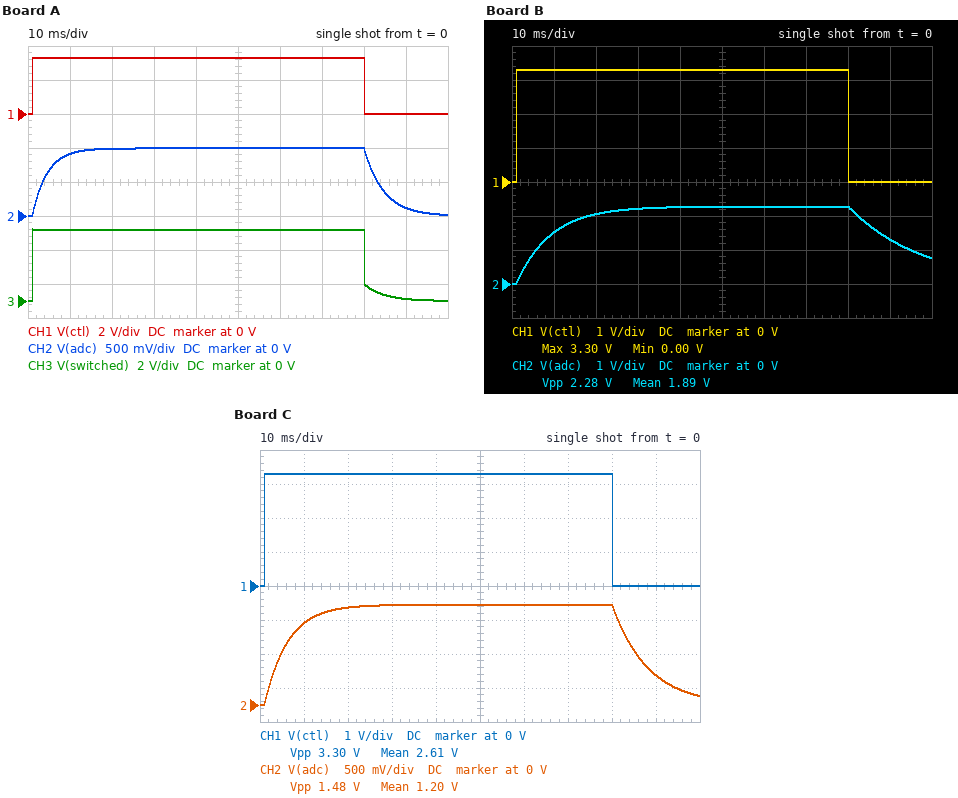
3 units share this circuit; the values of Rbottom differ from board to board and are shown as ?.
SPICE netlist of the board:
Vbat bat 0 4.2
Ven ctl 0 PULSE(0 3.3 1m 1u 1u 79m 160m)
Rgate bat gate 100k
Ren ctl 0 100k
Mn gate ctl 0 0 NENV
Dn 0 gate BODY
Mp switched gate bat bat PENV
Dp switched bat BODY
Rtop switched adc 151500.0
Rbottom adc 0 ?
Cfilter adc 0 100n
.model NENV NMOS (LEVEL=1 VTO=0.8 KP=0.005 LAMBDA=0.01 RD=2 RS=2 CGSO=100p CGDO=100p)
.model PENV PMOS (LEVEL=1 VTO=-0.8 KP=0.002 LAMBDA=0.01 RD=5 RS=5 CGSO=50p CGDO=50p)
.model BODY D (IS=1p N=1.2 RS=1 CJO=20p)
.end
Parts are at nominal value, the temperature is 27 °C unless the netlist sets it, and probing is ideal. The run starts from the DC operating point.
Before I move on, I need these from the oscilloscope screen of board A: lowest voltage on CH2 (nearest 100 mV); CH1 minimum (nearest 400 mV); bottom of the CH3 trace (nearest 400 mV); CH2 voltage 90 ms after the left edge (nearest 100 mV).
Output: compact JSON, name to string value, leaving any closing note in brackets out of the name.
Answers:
{"lowest voltage on CH2": "0 V", "CH1 minimum": "0 V", "bottom of the CH3 trace": "0 V", "CH2 voltage 90 ms after the left edge": "100 mV"}
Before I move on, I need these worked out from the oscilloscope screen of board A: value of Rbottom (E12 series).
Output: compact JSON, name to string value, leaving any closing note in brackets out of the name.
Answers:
{"value of Rbottom": "47 kΩ"}
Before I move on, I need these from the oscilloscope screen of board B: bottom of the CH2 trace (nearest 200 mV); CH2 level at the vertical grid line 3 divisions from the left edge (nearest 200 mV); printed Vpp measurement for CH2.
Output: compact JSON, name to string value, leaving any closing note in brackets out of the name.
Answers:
{"bottom of the CH2 trace": "0 V", "CH2 level at the vertical grid line 3 divisions from the left edge": "2.2 V", "printed Vpp measurement for CH2": "2.28 V"}
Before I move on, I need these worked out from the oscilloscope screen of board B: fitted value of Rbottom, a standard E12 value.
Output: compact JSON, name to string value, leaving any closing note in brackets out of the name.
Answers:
{"fitted value of Rbottom, a standard E12 value": "180 kΩ"}
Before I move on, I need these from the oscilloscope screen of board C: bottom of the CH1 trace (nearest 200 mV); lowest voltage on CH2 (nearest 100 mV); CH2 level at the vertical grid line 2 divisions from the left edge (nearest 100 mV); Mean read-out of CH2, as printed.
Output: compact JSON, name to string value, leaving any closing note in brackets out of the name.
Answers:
{"bottom of the CH1 trace": "0 V", "lowest voltage on CH2": "0 V", "CH2 level at the vertical grid line 2 divisions from the left edge": "1.4 V", "Mean read-out of CH2, as printed": "1.20 V"}
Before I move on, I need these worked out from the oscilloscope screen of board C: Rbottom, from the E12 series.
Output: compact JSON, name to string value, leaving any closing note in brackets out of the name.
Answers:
{"Rbottom, from the E12 series": "82 kΩ"}
